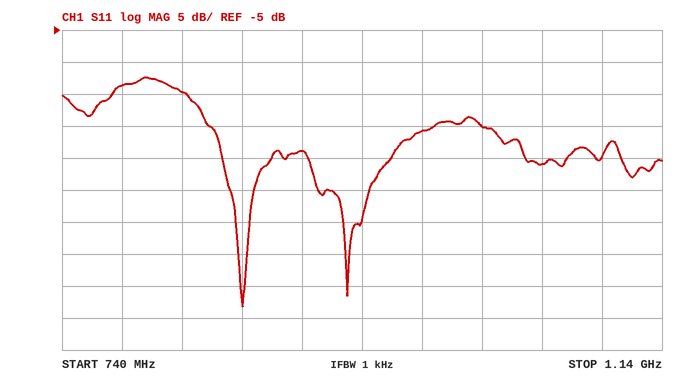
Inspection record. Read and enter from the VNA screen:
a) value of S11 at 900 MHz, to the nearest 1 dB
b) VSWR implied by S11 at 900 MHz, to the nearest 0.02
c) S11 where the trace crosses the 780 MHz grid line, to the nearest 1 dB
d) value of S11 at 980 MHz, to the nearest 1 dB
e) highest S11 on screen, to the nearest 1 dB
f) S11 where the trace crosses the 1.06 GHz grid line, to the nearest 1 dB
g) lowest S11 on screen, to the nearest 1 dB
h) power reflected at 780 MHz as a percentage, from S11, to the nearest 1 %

-24 dB
1.14
-14 dB
-21 dB
-12 dB
-26 dB
-48 dB
4 %
